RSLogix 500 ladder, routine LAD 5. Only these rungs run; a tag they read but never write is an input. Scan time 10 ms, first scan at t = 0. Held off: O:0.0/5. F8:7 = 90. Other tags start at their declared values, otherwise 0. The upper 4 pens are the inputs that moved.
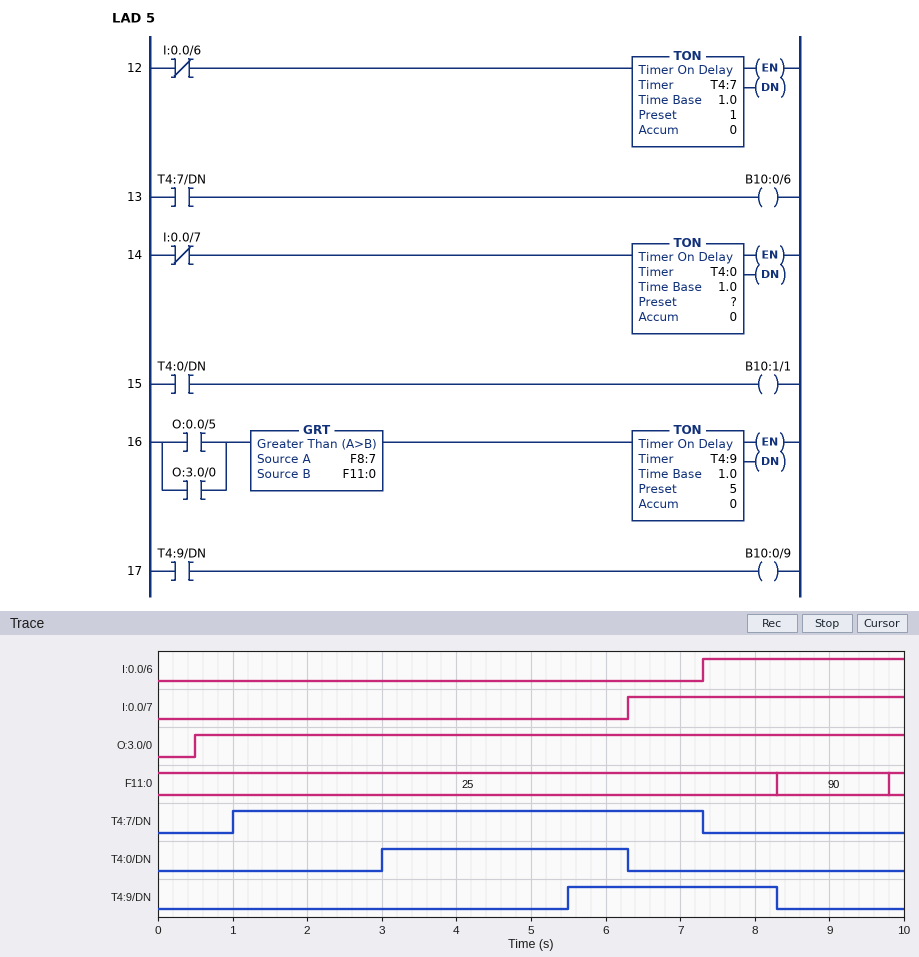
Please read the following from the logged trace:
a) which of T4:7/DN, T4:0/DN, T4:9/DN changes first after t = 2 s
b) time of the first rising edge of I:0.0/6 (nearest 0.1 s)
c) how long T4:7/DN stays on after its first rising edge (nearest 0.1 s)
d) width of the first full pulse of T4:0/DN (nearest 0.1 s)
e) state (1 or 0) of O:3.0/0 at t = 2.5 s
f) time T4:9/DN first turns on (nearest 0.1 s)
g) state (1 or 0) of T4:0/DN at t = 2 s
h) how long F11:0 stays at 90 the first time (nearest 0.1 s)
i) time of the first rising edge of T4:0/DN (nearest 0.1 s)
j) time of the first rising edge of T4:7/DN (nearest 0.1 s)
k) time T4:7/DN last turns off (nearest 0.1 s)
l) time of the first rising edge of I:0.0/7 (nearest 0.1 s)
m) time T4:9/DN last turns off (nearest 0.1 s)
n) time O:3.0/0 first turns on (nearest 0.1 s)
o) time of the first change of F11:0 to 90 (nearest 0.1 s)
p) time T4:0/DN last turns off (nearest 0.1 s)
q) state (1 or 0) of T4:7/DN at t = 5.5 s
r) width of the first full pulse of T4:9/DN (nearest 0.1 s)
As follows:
T4:0/DN
7.3 s
6.3 s
3.3 s
1
5.5 s
0
1.5 s
3.0 s
1.0 s
7.3 s
6.3 s
8.3 s
0.5 s
8.3 s
6.3 s
1
2.8 s
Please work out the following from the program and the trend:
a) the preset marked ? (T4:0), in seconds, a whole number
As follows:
3 s
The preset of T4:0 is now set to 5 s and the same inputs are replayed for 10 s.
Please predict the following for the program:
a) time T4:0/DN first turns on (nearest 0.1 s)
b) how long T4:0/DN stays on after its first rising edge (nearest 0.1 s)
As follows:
5.0 s
1.3 s
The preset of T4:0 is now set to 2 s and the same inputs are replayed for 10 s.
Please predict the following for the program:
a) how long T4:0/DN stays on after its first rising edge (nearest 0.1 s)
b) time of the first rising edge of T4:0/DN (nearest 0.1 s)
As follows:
4.3 s
2.0 s
